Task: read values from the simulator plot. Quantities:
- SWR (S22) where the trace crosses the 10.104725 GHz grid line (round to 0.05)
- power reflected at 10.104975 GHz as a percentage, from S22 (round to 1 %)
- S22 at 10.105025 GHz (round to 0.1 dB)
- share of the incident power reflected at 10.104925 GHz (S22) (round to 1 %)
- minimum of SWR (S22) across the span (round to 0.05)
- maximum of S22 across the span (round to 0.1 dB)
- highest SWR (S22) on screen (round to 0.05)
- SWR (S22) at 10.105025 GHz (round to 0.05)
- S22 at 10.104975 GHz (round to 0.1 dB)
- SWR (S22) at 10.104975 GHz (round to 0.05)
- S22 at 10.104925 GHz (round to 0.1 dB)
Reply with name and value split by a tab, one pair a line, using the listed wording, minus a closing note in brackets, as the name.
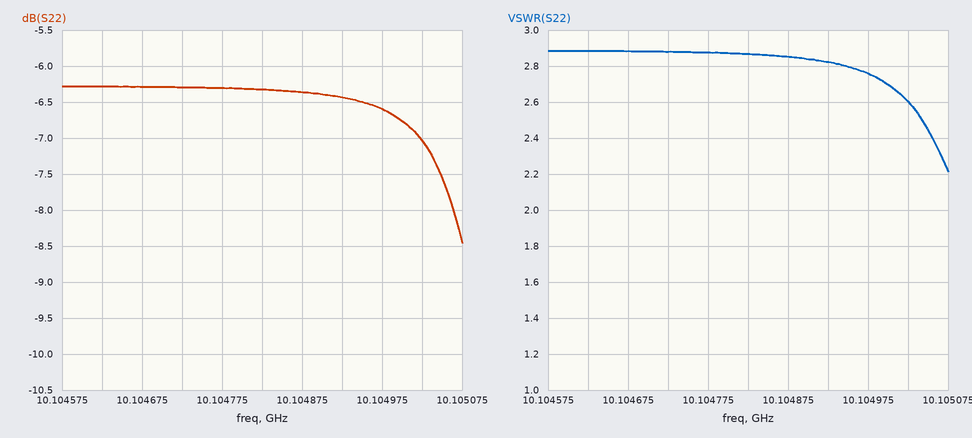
SWR (S22) where the trace crosses the 10.104725 GHz grid line	2.90
power reflected at 10.104975 GHz as a percentage, from S22	22 %
S22 at 10.105025 GHz	-7.0 dB
share of the incident power reflected at 10.104925 GHz (S22)	23 %
minimum of SWR (S22) across the span	2.20
maximum of S22 across the span	-6.3 dB
highest SWR (S22) on screen	2.90
SWR (S22) at 10.105025 GHz	2.60
S22 at 10.104975 GHz	-6.6 dB
SWR (S22) at 10.104975 GHz	2.75
S22 at 10.104925 GHz	-6.4 dB
